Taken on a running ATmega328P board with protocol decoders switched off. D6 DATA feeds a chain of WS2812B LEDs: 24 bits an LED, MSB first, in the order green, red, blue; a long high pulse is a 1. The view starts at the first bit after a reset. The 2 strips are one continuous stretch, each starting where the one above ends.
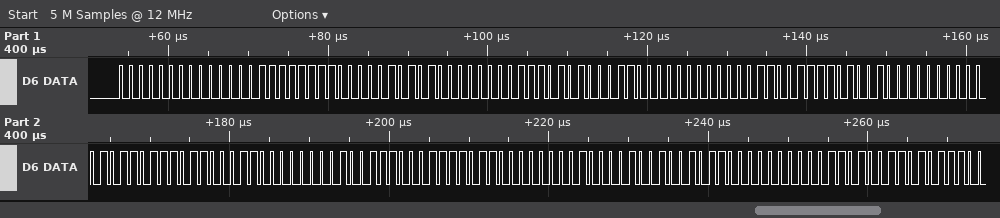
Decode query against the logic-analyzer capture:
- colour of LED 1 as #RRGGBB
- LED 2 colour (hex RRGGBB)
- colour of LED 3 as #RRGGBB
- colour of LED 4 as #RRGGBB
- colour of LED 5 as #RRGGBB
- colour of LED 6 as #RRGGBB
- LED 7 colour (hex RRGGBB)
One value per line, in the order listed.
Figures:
#0300FC
#0015EA
#0030CF
#0048B7
#00639C
#007B84
#009669
